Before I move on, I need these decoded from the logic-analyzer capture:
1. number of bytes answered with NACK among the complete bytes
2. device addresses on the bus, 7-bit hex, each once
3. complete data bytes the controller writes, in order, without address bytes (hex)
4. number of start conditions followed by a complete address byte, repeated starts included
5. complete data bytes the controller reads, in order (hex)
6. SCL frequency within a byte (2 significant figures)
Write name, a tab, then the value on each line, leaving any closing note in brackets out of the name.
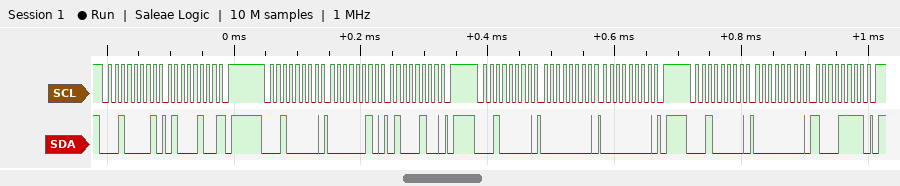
number of bytes answered with NACK among the complete bytes	1
device addresses on the bus, 7-bit hex, each once	0x10
complete data bytes the controller writes, in order, without address bytes	02 44 00 00 00 8F
number of start conditions followed by a complete address byte, repeated starts included	4
complete data bytes the controller reads, in order	44
SCL frequency within a byte	100 kHz
